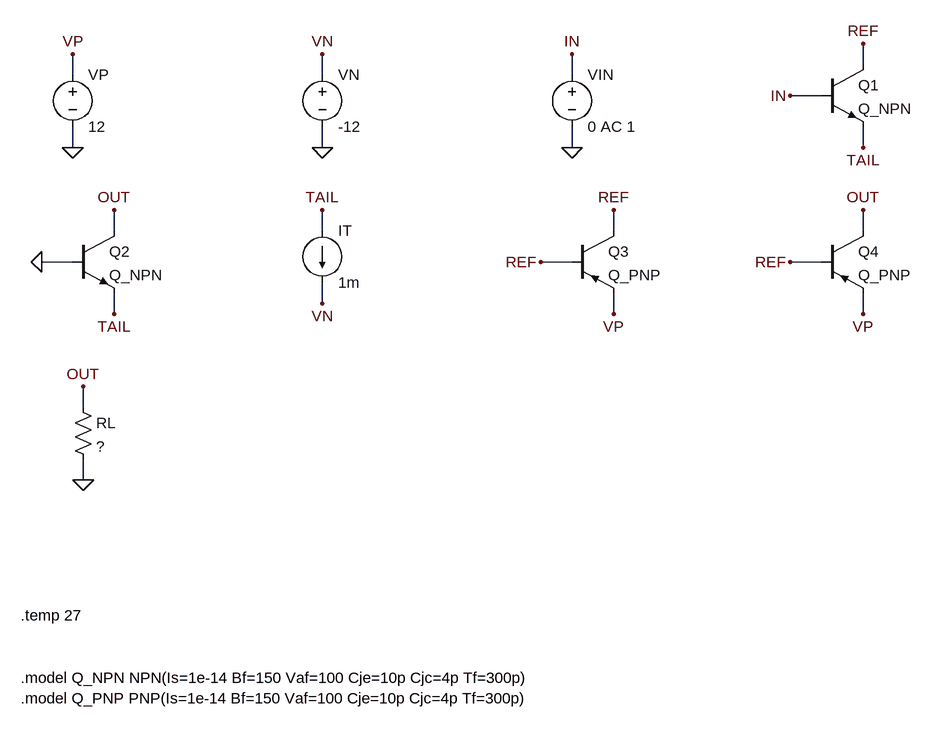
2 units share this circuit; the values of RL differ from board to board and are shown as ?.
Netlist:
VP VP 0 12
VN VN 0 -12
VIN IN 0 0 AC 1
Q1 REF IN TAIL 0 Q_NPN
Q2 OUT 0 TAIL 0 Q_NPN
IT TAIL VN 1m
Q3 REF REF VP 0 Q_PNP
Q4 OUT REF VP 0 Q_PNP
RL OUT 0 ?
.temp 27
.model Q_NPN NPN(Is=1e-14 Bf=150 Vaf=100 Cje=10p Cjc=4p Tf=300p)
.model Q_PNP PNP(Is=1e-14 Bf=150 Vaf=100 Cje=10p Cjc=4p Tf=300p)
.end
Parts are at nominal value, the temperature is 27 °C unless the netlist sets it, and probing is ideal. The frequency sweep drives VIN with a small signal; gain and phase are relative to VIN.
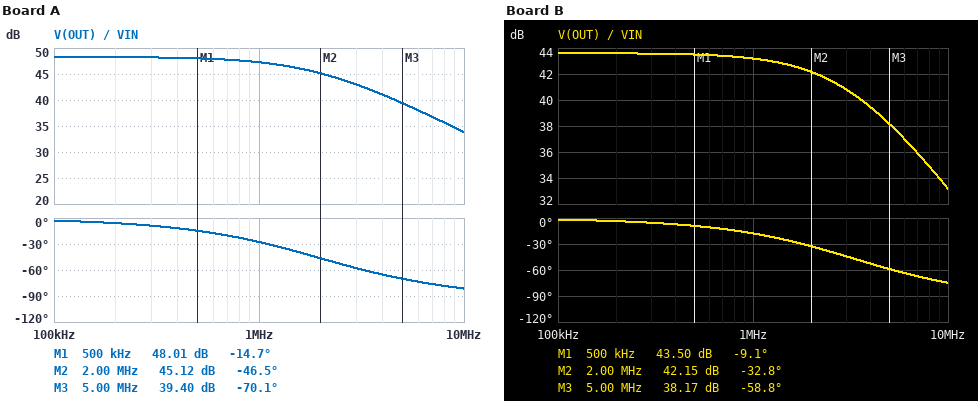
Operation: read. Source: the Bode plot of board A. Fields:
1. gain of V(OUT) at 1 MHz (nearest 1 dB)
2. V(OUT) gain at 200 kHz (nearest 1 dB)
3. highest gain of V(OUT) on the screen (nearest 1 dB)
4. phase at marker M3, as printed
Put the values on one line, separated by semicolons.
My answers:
47 dB; 48 dB; 48 dB; -70.1 deg
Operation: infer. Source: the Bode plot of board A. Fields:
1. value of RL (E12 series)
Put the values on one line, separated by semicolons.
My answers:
15 kΩ
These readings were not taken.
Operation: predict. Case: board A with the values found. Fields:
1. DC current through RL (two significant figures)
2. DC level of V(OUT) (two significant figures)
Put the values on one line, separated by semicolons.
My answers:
91 µA; 1.4 V
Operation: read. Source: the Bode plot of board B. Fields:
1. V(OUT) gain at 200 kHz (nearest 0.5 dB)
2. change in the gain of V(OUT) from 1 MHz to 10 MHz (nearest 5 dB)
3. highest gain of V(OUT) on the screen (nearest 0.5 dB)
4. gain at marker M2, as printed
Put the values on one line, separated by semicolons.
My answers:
43.5 dB; -10 dB; 43.5 dB; 42.15 dB
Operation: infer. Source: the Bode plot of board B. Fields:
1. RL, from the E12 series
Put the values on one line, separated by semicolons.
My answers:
8.2 kΩ
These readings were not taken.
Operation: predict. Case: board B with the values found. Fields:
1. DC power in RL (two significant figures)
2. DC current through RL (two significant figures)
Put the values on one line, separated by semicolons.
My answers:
77 µW; 97 µA
